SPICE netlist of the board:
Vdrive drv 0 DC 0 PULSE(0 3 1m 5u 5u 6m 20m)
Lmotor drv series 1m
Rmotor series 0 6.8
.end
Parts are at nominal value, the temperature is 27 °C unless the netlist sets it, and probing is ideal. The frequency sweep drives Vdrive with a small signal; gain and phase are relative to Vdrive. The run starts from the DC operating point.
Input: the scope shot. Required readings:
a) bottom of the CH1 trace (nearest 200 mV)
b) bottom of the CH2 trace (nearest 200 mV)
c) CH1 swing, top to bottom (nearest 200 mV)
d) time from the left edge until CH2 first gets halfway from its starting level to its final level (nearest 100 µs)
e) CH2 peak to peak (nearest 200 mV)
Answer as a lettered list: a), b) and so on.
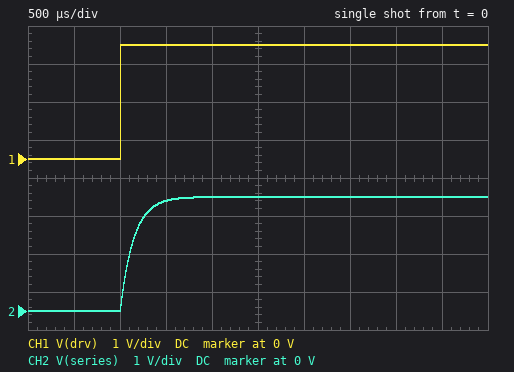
a) 0 V
b) 0 V
c) 3.0 V
d) 1.1 ms
e) 3.0 V
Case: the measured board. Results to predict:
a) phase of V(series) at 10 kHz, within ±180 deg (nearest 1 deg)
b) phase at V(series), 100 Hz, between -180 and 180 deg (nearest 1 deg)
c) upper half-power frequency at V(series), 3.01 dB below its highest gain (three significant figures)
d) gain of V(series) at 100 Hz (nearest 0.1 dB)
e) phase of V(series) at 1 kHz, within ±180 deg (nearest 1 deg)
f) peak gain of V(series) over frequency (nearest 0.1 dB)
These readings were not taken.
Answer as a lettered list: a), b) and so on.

a) -84 deg
b) -5 deg
c) 1.08 kHz
d) 0 dB
e) -43 deg
f) 0 dB
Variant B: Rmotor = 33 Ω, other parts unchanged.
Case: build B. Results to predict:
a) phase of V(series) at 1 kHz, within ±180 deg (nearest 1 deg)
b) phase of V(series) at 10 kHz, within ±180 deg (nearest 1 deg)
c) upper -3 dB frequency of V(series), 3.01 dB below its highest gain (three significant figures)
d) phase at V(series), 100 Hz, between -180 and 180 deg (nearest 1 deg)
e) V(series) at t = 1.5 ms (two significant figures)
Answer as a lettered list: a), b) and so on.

a) -11 deg
b) -62 deg
c) 5.25 kHz
d) -1 deg
e) 3.0 V
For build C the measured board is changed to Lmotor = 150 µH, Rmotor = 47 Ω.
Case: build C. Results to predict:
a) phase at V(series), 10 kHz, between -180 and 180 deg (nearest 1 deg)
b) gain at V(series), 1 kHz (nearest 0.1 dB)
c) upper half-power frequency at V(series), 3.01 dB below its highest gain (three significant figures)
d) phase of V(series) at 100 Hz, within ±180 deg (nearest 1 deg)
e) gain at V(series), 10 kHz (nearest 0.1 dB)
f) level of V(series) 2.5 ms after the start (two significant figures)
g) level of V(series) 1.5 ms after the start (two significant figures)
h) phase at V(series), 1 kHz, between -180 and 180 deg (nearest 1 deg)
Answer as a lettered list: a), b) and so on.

a) -11 deg
b) 0 dB
c) 49.9 kHz
d) 0 deg
e) -0.2 dB
f) 3.0 V
g) 3.0 V
h) -1 deg
